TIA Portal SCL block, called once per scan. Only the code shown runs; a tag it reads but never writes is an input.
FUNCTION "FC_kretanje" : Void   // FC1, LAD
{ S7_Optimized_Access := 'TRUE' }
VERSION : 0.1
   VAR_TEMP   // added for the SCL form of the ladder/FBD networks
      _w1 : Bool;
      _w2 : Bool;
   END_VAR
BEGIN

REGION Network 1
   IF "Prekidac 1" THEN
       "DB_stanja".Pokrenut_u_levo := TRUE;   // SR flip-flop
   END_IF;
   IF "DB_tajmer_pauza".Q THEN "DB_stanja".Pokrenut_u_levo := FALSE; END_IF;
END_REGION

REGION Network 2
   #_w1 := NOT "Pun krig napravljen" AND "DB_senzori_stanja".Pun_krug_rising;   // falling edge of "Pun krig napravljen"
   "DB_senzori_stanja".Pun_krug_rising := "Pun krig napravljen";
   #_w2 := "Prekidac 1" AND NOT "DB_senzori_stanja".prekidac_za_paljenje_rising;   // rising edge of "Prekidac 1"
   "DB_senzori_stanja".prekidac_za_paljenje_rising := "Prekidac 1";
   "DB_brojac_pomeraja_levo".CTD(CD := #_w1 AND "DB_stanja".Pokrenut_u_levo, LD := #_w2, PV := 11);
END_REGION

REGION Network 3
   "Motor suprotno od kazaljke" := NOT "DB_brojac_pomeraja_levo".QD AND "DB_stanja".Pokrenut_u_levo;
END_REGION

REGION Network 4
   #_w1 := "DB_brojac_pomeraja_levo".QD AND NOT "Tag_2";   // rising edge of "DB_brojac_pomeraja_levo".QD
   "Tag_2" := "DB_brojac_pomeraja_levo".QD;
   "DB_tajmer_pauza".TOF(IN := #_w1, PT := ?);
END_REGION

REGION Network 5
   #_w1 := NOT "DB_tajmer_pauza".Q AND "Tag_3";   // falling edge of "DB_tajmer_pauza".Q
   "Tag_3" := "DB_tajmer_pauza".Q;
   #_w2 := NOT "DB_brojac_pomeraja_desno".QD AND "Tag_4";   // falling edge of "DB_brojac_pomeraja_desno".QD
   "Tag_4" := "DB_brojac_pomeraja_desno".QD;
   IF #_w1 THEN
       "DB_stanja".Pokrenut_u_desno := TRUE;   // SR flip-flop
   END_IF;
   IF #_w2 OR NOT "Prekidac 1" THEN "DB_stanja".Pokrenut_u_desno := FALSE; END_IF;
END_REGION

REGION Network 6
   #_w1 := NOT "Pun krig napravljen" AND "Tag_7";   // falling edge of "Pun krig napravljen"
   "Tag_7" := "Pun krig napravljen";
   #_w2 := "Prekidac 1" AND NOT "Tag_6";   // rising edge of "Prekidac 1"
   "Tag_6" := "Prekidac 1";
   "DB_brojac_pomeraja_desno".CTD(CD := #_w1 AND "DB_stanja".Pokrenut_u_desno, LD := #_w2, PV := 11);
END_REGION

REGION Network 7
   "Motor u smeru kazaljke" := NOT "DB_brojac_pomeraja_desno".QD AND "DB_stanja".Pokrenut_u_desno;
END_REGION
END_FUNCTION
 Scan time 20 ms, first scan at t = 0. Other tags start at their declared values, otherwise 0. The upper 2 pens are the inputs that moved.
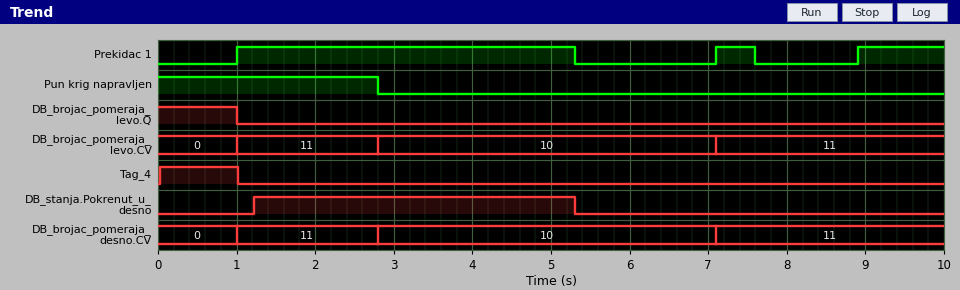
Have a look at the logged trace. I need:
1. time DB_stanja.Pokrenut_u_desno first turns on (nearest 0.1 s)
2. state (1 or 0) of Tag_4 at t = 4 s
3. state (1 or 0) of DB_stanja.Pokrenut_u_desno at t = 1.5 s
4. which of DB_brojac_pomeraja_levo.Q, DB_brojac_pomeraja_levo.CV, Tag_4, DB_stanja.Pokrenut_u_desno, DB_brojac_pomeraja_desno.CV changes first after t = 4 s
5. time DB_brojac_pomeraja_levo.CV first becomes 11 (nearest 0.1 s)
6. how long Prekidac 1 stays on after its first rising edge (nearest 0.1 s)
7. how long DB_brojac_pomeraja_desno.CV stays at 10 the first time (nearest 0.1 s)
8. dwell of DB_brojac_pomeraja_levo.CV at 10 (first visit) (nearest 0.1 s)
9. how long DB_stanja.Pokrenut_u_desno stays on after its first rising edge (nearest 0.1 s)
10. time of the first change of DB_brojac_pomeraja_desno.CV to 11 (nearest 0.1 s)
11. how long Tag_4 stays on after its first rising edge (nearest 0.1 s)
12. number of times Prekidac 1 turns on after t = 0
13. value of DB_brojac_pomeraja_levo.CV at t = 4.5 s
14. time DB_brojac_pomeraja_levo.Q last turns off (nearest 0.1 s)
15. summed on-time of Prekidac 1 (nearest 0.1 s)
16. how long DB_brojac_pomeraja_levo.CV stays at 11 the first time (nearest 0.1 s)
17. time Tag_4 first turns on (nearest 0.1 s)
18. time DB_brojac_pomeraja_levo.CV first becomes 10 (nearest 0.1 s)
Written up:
1.2 s
0
1
DB_stanja.Pokrenut_u_desno
1.0 s
4.3 s
4.3 s
4.3 s
4.1 s
1.0 s
1.0 s
3
10
1.0 s
5.9 s
1.8 s
0.0 s
2.8 s
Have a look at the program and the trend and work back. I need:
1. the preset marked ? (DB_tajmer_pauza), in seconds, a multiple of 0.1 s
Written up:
1.2 s
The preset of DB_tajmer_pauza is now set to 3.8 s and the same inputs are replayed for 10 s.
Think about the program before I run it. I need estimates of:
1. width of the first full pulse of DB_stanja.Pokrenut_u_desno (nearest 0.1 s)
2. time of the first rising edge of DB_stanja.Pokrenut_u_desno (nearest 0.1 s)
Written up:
1.5 s
3.8 s
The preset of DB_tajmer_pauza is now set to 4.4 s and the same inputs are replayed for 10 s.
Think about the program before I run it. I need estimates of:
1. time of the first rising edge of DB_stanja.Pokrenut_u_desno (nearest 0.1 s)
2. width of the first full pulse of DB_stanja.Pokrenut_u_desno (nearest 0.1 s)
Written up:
4.4 s
0.9 s
